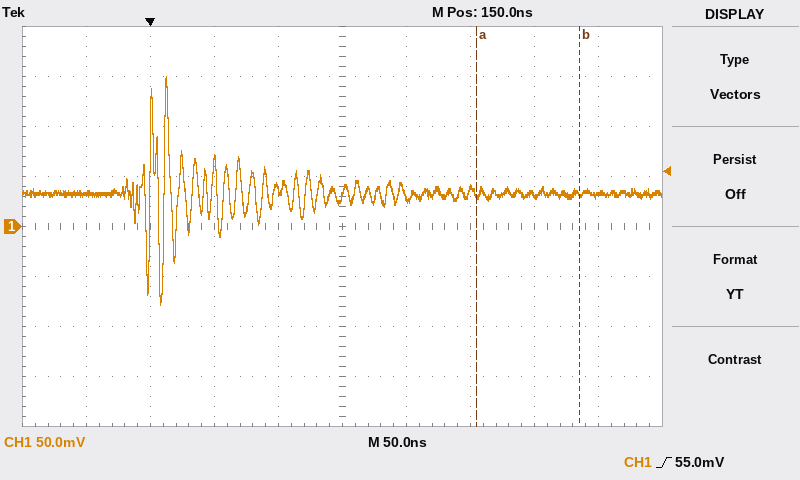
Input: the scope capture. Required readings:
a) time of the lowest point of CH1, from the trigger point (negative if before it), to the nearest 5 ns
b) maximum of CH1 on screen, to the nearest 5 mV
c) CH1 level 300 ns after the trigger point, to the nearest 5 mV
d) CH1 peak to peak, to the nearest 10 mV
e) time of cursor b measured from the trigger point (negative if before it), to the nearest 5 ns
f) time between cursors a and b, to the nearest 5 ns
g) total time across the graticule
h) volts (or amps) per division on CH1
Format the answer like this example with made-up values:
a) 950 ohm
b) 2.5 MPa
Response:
a) +10 ns
b) 150 mV
c) 30 mV
d) 230 mV
e) +335 ns
f) 80 ns
g) 500 ns
h) 50 mV
